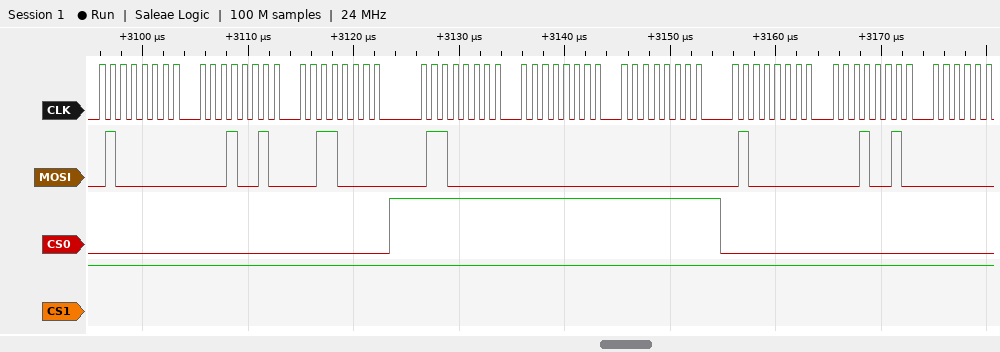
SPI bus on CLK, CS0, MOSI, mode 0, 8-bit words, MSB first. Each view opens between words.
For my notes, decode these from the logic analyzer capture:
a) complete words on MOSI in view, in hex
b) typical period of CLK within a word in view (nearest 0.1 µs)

40, 12, 30, 60, 00, 00, 40, 12
1 µs
